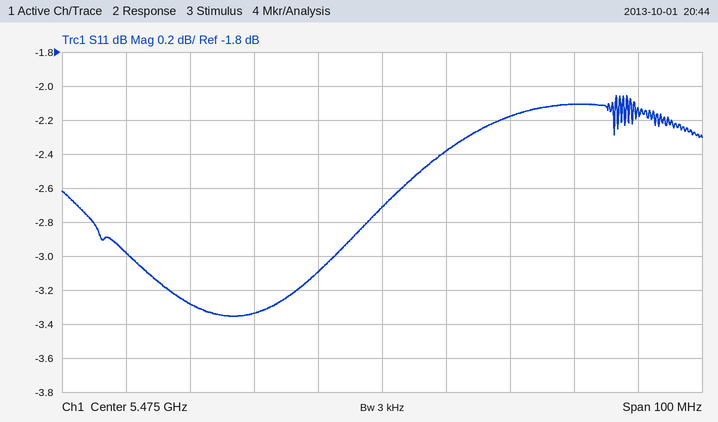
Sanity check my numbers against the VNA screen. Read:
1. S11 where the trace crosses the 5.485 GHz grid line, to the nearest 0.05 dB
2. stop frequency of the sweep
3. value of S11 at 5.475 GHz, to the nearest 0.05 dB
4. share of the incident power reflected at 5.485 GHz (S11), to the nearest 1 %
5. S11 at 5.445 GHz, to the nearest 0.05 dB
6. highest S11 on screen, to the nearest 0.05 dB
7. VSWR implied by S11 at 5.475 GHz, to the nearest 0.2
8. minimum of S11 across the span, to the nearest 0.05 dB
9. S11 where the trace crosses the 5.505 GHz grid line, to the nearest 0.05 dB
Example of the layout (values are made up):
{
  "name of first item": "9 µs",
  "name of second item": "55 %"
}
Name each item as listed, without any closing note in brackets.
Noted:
{
  "S11 where the trace crosses the 5.485 GHz grid line, to the nearest 0.05 dB": "-2.40 dB",
  "stop frequency of the sweep": "5.525 GHz",
  "value of S11 at 5.475 GHz, to the nearest 0.05 dB": "-2.70 dB",
  "share of the incident power reflected at 5.485 GHz (S11), to the nearest 1 %": "58 %",
  "S11 at 5.445 GHz, to the nearest 0.05 dB": "-3.30 dB",
  "highest S11 on screen, to the nearest 0.05 dB": "-2.05 dB",
  "VSWR implied by S11 at 5.475 GHz, to the nearest 0.2": "6.4",
  "minimum of S11 across the span, to the nearest 0.05 dB": "-3.35 dB",
  "S11 where the trace crosses the 5.505 GHz grid line, to the nearest 0.05 dB": "-2.10 dB"
}
